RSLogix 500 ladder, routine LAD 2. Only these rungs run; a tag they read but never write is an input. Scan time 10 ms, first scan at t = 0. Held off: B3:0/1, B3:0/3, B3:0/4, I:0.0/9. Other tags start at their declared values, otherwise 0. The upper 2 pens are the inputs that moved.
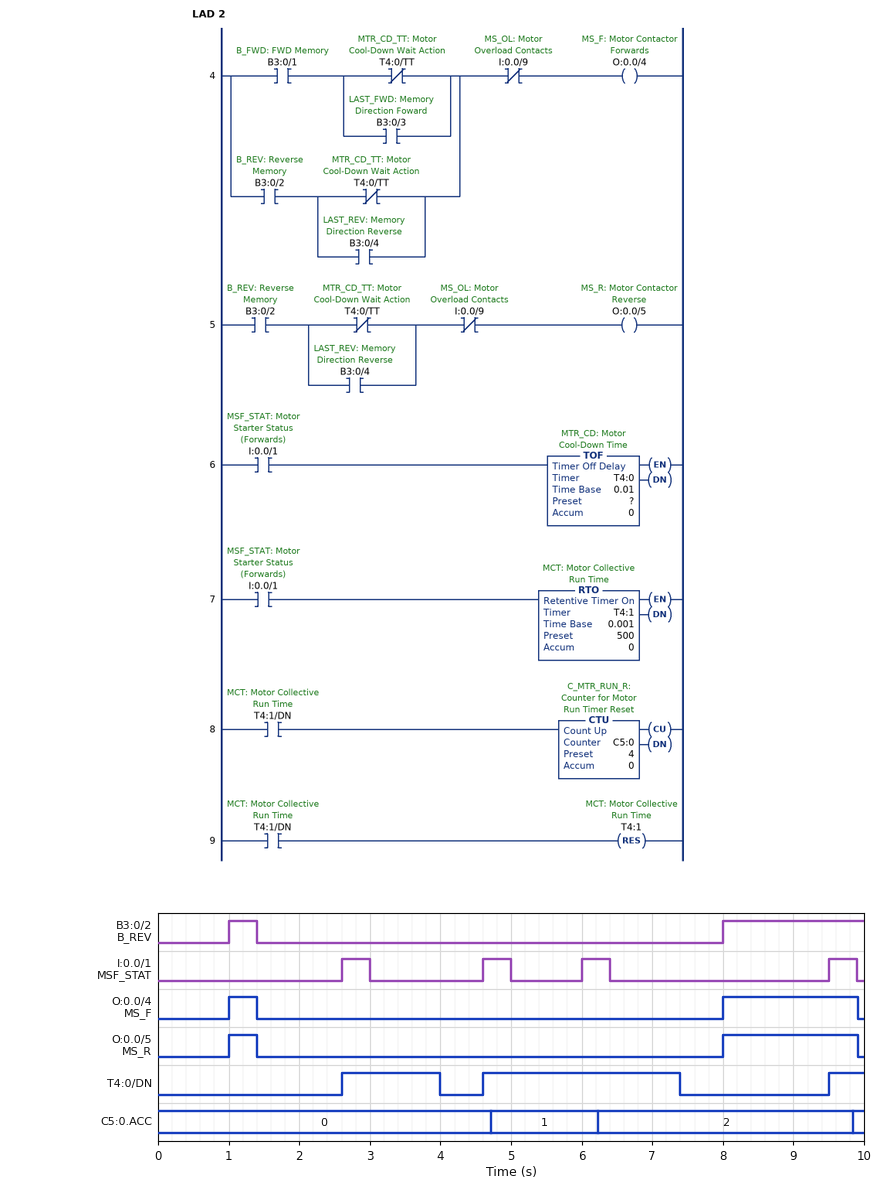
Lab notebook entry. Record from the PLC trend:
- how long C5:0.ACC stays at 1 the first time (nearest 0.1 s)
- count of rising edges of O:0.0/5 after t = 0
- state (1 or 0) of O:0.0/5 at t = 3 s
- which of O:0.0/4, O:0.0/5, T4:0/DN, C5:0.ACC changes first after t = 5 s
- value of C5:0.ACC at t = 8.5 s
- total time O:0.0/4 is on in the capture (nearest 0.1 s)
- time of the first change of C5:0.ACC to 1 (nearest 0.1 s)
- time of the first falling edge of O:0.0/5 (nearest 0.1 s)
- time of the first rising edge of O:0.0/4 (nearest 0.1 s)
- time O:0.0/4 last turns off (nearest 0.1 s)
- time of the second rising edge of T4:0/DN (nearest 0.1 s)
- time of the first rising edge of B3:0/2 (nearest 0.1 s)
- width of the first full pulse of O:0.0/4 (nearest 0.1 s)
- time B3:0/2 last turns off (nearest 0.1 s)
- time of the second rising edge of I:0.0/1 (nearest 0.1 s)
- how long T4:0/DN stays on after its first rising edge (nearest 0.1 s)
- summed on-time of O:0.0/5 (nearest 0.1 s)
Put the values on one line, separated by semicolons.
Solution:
1.5 s; 2; 0; C5:0.ACC; 2; 2.3 s; 4.7 s; 1.4 s; 1.0 s; 9.9 s; 4.6 s; 1.0 s; 0.4 s; 1.4 s; 4.6 s; 1.4 s; 2.3 s
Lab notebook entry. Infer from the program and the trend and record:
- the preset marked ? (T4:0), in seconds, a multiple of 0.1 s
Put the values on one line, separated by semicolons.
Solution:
1.0 s
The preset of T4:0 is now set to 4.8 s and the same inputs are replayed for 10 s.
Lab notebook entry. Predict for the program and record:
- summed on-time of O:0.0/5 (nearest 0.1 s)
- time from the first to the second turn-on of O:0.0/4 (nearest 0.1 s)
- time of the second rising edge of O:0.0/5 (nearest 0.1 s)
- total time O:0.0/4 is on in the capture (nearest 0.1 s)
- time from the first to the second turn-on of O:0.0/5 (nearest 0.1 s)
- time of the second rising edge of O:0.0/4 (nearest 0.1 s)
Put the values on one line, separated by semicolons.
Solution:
0.8 s; 8.5 s; 9.5 s; 0.8 s; 8.5 s; 9.5 s
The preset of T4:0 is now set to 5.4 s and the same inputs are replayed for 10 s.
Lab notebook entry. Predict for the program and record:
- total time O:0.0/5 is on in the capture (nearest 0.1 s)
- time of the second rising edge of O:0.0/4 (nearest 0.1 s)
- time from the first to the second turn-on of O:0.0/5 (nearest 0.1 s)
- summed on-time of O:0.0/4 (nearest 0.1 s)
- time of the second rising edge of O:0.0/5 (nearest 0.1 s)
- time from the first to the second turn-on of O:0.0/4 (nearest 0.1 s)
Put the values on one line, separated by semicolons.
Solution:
0.8 s; 9.5 s; 8.5 s; 0.8 s; 9.5 s; 8.5 s
